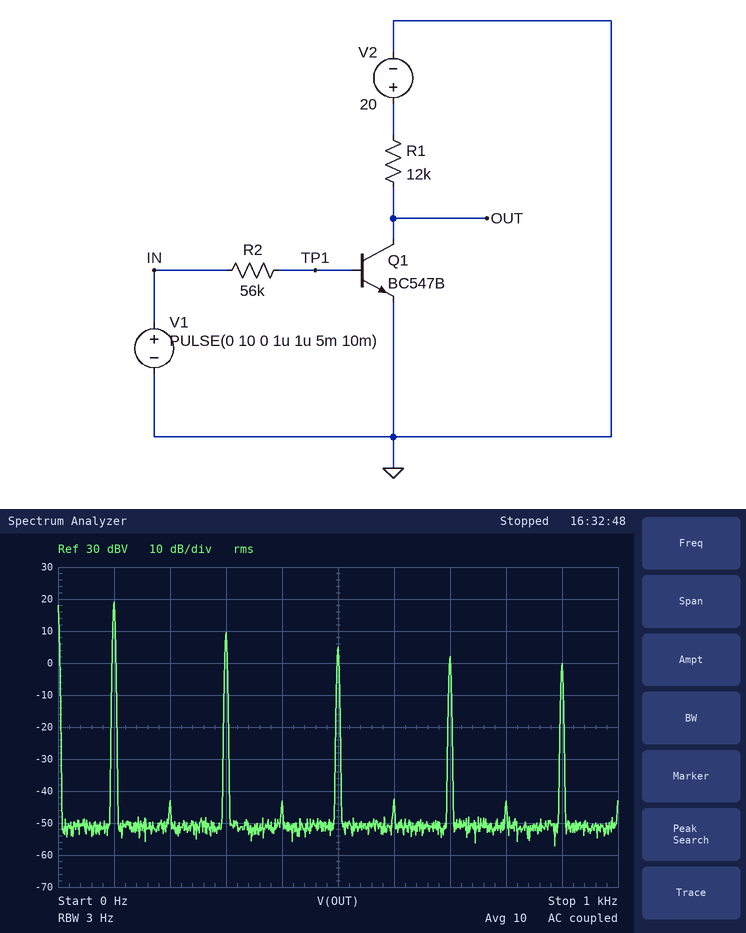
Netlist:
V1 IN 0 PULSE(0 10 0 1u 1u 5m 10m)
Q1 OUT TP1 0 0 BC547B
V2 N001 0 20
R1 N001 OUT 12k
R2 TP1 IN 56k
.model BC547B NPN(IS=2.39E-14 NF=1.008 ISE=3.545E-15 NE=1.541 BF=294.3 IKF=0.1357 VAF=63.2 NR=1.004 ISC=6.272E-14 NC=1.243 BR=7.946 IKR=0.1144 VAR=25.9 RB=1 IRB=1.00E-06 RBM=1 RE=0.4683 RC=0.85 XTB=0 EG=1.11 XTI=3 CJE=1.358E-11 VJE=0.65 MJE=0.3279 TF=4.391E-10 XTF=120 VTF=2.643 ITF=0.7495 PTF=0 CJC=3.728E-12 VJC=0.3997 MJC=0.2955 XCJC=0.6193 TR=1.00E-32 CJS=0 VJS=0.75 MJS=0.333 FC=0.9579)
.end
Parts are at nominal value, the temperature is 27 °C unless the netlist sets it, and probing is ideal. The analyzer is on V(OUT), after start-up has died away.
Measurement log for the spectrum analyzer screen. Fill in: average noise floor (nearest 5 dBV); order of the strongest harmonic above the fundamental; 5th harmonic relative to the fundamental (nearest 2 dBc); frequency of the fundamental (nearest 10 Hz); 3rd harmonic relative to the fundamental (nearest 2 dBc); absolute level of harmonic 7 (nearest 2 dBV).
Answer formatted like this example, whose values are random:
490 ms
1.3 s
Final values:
-50 dBV
3
-14 dBc
100 Hz
-10 dBc
2 dBV
